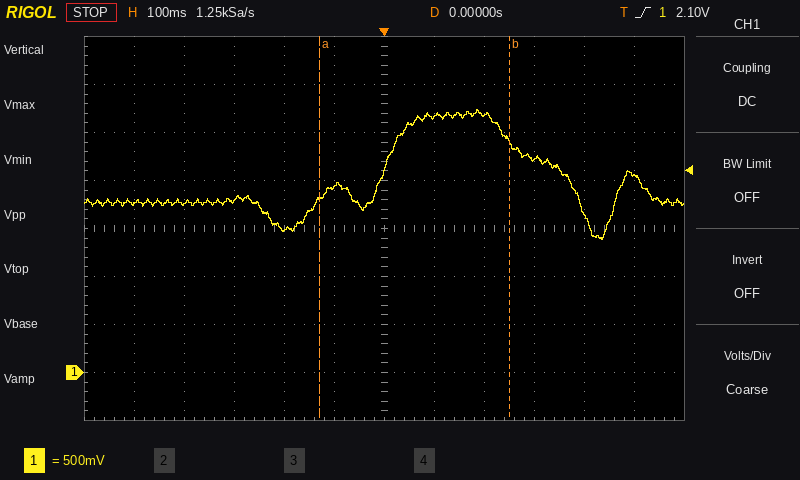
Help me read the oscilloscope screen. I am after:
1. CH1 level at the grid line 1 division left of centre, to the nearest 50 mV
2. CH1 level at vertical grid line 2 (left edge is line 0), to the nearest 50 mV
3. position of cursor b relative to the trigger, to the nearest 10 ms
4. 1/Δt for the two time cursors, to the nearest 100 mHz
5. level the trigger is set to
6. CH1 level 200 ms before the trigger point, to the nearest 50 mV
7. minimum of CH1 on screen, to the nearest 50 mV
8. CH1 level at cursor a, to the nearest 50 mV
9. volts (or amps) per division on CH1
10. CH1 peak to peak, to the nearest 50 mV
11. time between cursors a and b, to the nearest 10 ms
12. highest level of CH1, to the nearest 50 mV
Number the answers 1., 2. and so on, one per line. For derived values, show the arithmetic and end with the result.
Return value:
1. 1.95 V
2. 1.75 V
3. +250 ms
4. 1 / 380 ms ≈ 2.6 Hz
5. 2.10 V
6. 1.50 V
7. 1.40 V
8. 1.80 V
9. 500 mV
10. 2.75 V − (1.40 V) = 1.35 V
11. 380 ms
12. 2.75 V
